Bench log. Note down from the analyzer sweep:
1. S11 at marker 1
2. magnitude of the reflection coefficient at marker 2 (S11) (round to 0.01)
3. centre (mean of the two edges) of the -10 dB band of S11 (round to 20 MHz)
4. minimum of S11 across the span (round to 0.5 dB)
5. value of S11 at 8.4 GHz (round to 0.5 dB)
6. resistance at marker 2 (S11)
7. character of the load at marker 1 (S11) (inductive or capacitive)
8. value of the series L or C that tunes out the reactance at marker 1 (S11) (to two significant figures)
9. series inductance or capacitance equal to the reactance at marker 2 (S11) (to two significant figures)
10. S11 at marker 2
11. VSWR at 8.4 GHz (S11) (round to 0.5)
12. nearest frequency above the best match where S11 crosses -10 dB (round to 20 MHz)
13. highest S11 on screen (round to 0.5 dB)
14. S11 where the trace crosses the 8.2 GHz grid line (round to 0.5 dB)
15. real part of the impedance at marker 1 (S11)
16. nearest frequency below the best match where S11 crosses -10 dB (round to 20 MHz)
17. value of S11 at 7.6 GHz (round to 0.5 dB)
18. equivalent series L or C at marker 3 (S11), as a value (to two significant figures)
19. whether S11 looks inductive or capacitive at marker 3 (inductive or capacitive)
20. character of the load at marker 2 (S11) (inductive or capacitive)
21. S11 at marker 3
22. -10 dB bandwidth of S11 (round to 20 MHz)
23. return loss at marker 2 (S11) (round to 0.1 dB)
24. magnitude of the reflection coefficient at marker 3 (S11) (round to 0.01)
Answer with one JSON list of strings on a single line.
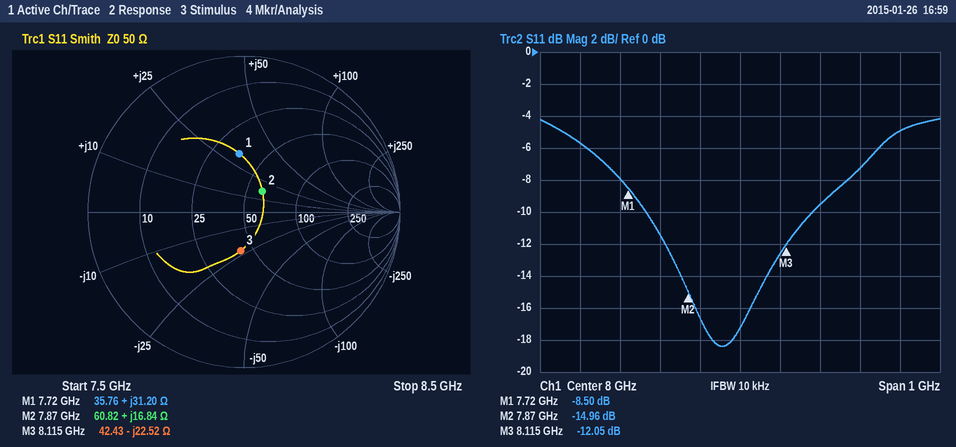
["-8.50 dB", "0.18", "7.98 GHz", "-18.5 dB", "-5.0 dB", "60.82 Ω", "inductive", "660 fF", "340 pH", "-14.96 dB", "3.5", "8.18 GHz", "-4.0 dB", "-9.5 dB", "35.76 Ω", "7.76 GHz", "-5.5 dB", "870 fF", "capacitive", "inductive", "-12.05 dB", "420 MHz", "15.0 dB", "0.25"]
